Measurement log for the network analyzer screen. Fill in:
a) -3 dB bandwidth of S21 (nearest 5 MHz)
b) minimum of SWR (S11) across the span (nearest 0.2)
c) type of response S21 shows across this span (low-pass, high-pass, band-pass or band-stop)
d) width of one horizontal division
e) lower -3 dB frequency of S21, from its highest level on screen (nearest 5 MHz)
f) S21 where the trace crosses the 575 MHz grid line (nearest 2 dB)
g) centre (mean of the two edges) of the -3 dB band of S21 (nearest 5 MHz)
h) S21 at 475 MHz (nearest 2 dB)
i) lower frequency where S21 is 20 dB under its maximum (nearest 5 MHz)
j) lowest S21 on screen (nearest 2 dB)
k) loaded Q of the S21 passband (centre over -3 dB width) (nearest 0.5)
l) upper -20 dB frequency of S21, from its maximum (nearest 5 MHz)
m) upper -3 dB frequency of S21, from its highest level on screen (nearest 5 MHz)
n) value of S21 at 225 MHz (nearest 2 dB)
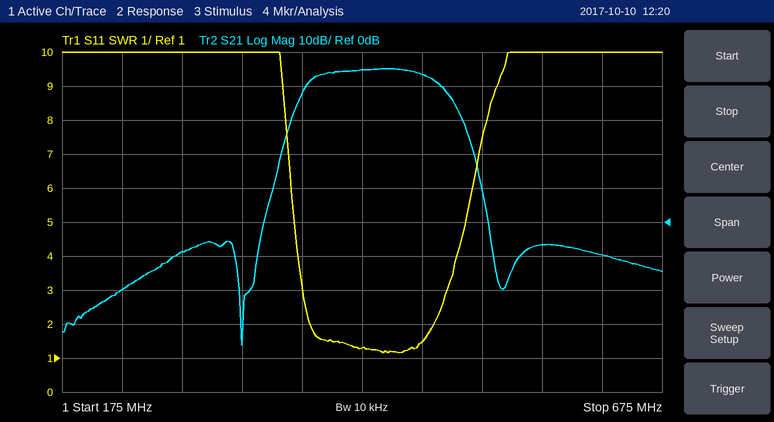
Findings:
100 MHz
1.2
band-pass
50 MHz
385 MHz
-6 dB
435 MHz
44 dB
360 MHz
-36 dB
4.5
515 MHz
485 MHz
-20 dB
